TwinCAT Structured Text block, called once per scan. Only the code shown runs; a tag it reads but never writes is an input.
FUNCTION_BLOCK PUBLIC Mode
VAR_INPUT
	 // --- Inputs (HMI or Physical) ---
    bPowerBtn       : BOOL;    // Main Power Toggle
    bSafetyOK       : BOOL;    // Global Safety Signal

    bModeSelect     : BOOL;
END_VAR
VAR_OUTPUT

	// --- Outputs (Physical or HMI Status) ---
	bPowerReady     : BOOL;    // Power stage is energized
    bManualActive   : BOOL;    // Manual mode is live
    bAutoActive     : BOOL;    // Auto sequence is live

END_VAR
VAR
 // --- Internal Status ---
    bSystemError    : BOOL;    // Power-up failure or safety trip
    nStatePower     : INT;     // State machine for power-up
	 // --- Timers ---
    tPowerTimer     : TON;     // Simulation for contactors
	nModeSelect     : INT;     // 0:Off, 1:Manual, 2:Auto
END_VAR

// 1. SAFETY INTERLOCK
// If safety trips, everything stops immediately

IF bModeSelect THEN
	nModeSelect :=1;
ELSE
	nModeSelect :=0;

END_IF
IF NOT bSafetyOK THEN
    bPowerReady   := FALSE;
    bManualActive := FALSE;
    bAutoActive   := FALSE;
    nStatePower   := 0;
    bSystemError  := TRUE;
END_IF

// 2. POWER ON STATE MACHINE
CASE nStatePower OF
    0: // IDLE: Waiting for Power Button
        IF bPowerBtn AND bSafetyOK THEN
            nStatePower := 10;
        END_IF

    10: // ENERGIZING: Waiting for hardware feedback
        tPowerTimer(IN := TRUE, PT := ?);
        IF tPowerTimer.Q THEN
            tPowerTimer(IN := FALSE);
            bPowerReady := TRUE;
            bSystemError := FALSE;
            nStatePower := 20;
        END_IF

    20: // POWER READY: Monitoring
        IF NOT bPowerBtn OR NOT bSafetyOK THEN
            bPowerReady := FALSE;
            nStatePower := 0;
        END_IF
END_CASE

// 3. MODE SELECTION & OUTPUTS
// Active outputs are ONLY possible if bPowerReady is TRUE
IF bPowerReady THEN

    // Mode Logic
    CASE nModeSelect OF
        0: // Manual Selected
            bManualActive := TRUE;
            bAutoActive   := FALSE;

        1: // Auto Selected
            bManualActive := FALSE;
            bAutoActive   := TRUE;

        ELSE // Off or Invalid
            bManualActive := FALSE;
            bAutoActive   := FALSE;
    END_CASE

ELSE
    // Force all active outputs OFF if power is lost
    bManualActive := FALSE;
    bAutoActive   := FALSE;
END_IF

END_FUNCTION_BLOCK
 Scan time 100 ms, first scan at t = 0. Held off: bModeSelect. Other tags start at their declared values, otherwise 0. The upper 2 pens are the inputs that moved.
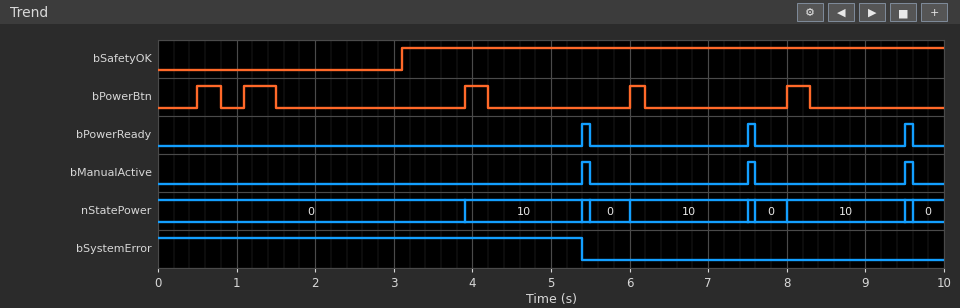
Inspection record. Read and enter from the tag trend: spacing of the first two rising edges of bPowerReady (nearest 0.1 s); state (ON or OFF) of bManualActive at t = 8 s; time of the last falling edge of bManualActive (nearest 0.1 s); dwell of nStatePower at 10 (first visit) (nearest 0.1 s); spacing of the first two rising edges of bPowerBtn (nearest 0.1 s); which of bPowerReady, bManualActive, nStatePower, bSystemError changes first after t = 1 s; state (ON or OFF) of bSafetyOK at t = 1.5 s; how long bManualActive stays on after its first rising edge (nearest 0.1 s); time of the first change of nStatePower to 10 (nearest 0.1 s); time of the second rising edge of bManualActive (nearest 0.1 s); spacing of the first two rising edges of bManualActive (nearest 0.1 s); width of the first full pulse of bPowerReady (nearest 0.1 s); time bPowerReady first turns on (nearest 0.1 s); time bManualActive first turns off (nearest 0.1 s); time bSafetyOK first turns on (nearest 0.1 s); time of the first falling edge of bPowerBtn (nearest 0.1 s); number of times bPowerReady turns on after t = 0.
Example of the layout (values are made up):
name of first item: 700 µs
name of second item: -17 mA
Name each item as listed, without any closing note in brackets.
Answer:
spacing of the first two rising edges of bPowerReady: 2.1 s
state (ON or OFF) of bManualActive at t = 8 s: OFF
time of the last falling edge of bManualActive: 9.6 s
dwell of nStatePower at 10 (first visit): 1.5 s
spacing of the first two rising edges of bPowerBtn: 0.6 s
which of bPowerReady, bManualActive, nStatePower, bSystemError changes first after t = 1 s: nStatePower
state (ON or OFF) of bSafetyOK at t = 1.5 s: OFF
how long bManualActive stays on after its first rising edge: 0.1 s
time of the first change of nStatePower to 10: 3.9 s
time of the second rising edge of bManualActive: 7.5 s
spacing of the first two rising edges of bManualActive: 2.1 s
width of the first full pulse of bPowerReady: 0.1 s
time bPowerReady first turns on: 5.4 s
time bManualActive first turns off: 5.5 s
time bSafetyOK first turns on: 3.1 s
time of the first falling edge of bPowerBtn: 0.8 s
number of times bPowerReady turns on after t = 0: 3
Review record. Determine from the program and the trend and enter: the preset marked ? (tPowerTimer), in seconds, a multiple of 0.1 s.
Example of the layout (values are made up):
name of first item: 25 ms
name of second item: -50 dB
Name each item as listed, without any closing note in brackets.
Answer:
the preset marked ? (tPowerTimer), in seconds, a multiple of 0.1 s: 1.4 s
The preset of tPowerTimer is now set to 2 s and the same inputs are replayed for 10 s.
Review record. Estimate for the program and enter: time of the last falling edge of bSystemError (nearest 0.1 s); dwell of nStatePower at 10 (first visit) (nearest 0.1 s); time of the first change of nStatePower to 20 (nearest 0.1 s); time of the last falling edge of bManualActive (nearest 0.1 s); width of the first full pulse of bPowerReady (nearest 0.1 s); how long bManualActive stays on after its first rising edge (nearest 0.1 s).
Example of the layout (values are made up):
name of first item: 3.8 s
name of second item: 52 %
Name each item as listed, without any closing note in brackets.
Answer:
time of the last falling edge of bSystemError: 6.0 s
dwell of nStatePower at 10 (first visit): 2.1 s
time of the first change of nStatePower to 20: 6.0 s
time of the last falling edge of bManualActive: 6.2 s
width of the first full pulse of bPowerReady: 0.2 s
how long bManualActive stays on after its first rising edge: 0.2 s
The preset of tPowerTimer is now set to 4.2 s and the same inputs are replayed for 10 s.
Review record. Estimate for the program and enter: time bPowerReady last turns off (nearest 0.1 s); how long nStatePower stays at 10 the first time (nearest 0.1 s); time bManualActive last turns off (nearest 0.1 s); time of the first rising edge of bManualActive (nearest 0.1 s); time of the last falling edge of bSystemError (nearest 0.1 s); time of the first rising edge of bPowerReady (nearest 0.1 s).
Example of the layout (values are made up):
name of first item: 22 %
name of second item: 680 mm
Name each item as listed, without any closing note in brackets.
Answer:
time bPowerReady last turns off: 8.3 s
how long nStatePower stays at 10 the first time: 4.3 s
time bManualActive last turns off: 8.3 s
time of the first rising edge of bManualActive: 8.2 s
time of the last falling edge of bSystemError: 8.2 s
time of the first rising edge of bPowerReady: 8.2 s
